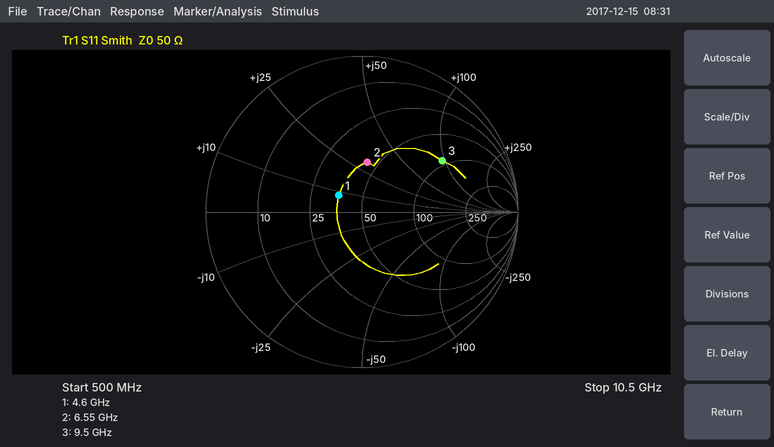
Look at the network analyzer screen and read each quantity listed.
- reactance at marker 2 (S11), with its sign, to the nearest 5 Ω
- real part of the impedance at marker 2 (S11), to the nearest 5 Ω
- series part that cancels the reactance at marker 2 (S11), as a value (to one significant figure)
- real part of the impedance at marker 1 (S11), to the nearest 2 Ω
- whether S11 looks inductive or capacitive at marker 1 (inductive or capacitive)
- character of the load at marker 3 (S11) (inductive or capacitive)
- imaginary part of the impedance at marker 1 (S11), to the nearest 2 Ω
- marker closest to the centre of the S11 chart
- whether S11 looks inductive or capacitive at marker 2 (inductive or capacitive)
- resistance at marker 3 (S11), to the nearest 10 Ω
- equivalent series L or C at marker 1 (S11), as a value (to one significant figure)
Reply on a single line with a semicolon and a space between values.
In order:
+30 Ω; 45 Ω; 800 fF; 36 Ω; inductive; inductive; +8 Ω; marker 1; inductive; 90 Ω; 300 pH
